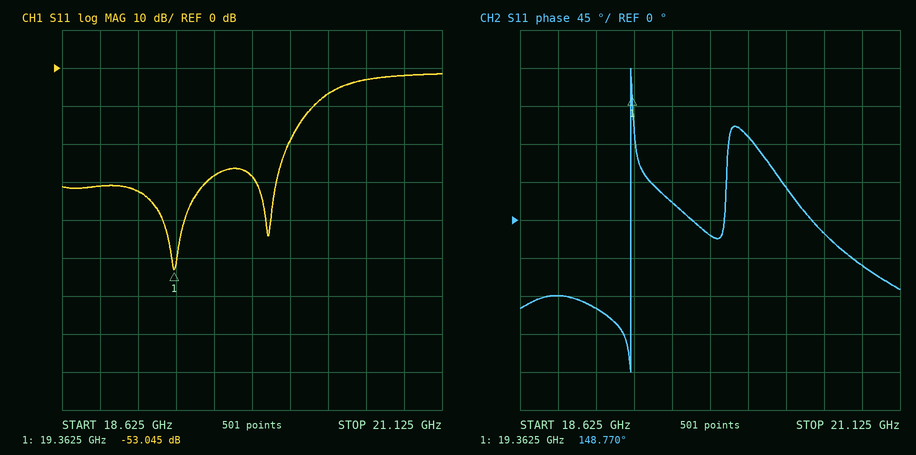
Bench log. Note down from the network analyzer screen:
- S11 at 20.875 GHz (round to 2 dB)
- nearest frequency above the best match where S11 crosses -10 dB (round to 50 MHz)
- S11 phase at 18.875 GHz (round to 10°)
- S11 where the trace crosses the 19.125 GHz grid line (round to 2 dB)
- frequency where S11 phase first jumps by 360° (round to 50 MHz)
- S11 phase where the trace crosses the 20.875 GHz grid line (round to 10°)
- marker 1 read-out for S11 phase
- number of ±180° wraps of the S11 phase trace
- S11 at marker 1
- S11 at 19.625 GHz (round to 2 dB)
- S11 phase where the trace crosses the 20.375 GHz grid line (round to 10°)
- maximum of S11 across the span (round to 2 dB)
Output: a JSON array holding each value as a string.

["-2 dB", "20.30 GHz", "-90°", "-32 dB", "19.35 GHz", "-50°", "148.770°", "1", "-53.045 dB", "-28 dB", "40°", "-2 dB"]
